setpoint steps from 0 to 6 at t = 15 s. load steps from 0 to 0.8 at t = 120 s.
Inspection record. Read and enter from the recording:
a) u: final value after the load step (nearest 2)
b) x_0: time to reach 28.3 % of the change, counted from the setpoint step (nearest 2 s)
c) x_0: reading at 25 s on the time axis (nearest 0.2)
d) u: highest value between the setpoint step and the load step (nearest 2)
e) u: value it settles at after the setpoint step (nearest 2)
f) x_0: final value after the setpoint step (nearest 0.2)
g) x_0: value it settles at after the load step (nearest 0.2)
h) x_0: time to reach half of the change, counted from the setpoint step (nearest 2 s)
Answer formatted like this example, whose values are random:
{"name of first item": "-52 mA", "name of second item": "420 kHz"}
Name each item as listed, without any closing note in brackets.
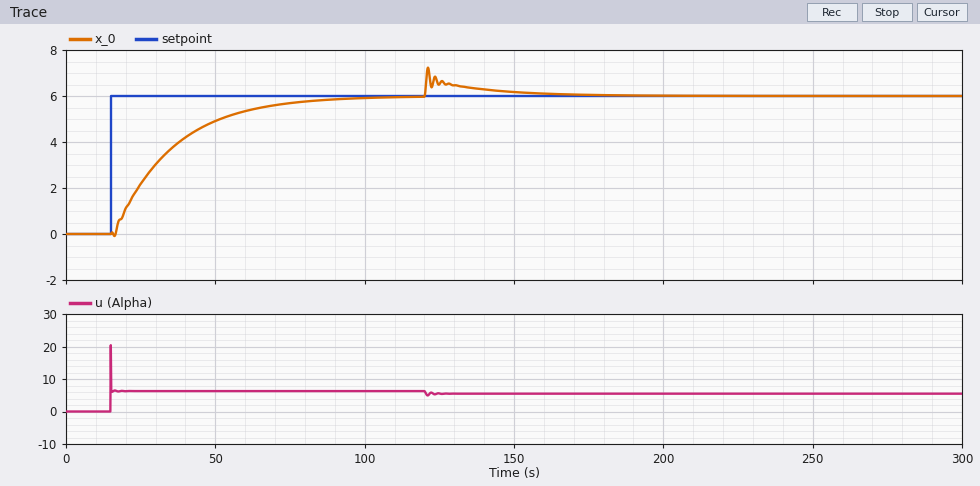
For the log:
{"u: final value after the load step": "6", "x_0: time to reach 28.3 % of the change, counted from the setpoint step": "8 s", "x_0: reading at 25 s on the time axis": "2.2", "u: highest value between the setpoint step and the load step": "20", "u: value it settles at after the setpoint step": "6", "x_0: final value after the setpoint step": "6.0", "x_0: value it settles at after the load step": "6.0", "x_0: time to reach half of the change, counted from the setpoint step": "14 s"}
